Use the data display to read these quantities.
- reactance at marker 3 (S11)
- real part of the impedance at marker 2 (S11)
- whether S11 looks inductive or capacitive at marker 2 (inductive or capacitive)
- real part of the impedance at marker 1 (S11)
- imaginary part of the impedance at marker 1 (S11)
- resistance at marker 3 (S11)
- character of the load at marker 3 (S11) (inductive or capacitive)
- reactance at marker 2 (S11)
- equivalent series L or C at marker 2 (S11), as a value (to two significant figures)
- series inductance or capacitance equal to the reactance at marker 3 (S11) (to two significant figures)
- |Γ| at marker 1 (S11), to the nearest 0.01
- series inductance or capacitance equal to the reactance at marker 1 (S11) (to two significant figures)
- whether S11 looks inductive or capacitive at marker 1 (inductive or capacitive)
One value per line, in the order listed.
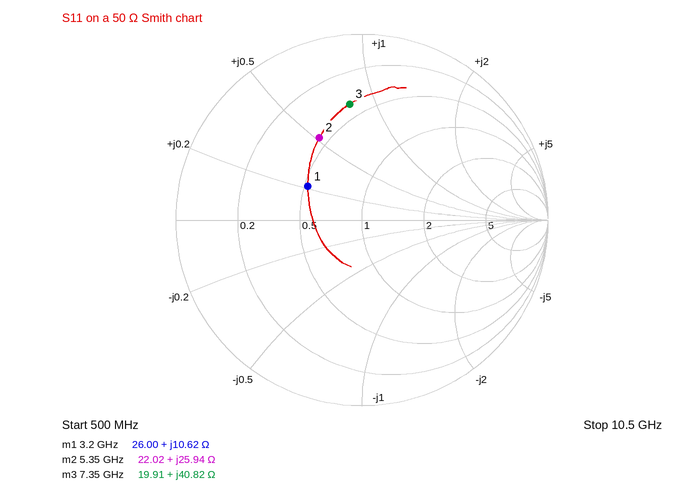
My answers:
+40.82 Ω
22.02 Ω
inductive
26.00 Ω
+10.62 Ω
19.91 Ω
inductive
+25.94 Ω
770 pH
880 pH
0.34
530 pH
inductive
